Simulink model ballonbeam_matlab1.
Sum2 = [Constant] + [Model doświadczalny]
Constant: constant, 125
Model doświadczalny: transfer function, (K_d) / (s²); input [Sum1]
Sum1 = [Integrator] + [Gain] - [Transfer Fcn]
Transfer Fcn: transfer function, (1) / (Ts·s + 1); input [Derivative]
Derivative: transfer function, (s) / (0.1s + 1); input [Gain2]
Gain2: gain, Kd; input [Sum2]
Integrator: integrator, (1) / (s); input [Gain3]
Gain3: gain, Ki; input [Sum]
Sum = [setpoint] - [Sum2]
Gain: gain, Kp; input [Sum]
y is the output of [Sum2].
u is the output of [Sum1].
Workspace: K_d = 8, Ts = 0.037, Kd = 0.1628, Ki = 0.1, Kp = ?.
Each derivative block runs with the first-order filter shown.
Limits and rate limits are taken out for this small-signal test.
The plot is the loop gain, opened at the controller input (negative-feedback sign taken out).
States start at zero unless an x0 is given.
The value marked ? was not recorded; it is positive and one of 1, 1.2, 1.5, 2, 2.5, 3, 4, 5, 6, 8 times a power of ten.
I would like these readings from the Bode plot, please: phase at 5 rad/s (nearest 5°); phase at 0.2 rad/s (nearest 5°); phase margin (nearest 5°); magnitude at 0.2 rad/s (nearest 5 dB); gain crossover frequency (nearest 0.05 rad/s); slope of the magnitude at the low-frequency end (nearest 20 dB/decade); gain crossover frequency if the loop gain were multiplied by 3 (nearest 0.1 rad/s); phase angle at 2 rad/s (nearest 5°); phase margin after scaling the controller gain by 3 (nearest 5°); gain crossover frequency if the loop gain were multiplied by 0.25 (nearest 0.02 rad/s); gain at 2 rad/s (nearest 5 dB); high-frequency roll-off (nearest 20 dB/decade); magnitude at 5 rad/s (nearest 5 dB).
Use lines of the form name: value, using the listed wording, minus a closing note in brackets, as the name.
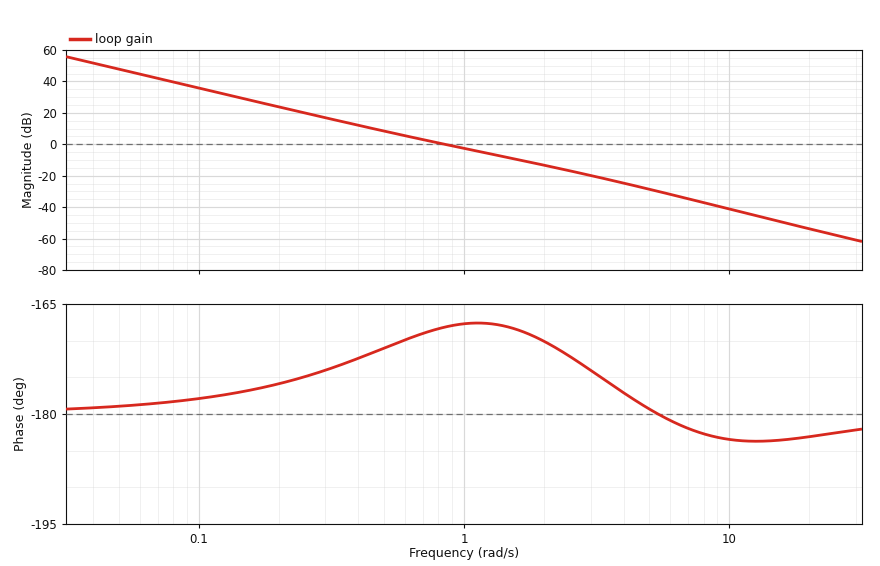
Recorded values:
phase at 5 rad/s: -180°
phase at 0.2 rad/s: -175°
phase margin: 10°
magnitude at 0.2 rad/s: 25 dB
gain crossover frequency: 0.85 rad/s
slope of the magnitude at the low-frequency end: -40 dB/decade
gain crossover frequency if the loop gain were multiplied by 3: 1.6 rad/s
phase angle at 2 rad/s: -170°
phase margin after scaling the controller gain by 3: 10°
gain crossover frequency if the loop gain were multiplied by 0.25: 0.40 rad/s
gain at 2 rad/s: -15 dB
high-frequency roll-off: -40 dB/decade
magnitude at 5 rad/s: -30 dB
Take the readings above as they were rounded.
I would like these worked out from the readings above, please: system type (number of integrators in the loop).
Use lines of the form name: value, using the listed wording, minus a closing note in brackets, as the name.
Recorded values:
system type: 2
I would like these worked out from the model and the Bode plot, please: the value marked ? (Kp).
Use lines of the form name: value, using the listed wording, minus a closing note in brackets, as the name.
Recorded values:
the value marked ?: 0.1
